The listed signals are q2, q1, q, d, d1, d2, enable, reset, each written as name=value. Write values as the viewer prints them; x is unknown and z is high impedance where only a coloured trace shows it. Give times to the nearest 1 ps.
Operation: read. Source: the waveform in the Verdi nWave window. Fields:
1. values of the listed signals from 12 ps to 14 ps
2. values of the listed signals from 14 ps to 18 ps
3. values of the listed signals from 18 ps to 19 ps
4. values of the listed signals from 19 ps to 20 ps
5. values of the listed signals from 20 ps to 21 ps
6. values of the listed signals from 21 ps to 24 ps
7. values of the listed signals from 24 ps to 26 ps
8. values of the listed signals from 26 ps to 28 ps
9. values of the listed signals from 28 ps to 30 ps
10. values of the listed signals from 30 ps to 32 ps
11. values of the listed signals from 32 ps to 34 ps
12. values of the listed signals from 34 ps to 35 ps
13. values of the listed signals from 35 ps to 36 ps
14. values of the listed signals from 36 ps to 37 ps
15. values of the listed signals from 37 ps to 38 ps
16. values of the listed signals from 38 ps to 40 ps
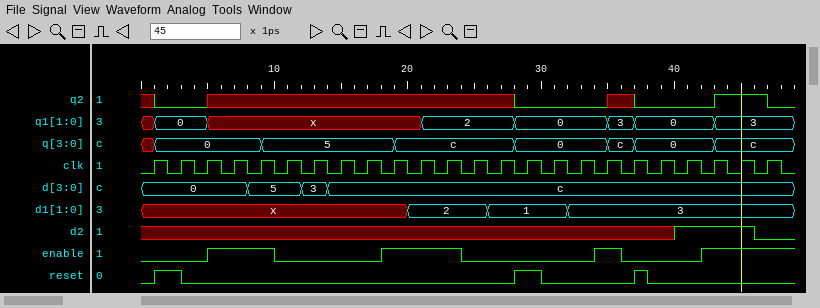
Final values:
q2=x, q1=x, q=5, d=3, d1=x, d2=x, enable=0, reset=0
q2=x, q1=x, q=5, d=c, d1=x, d2=x, enable=0, reset=0
q2=x, q1=x, q=5, d=c, d1=x, d2=x, enable=1, reset=0
q2=x, q1=x, q=c, d=c, d1=x, d2=x, enable=1, reset=0
q2=x, q1=x, q=c, d=c, d1=2, d2=x, enable=1, reset=0
q2=x, q1=2, q=c, d=c, d1=2, d2=x, enable=1, reset=0
q2=x, q1=2, q=c, d=c, d1=2, d2=x, enable=0, reset=0
q2=x, q1=2, q=c, d=c, d1=1, d2=x, enable=0, reset=0
q2=0, q1=0, q=0, d=c, d1=1, d2=x, enable=0, reset=1
q2=0, q1=0, q=0, d=c, d1=1, d2=x, enable=0, reset=0
q2=0, q1=0, q=0, d=c, d1=3, d2=x, enable=0, reset=0
q2=0, q1=0, q=0, d=c, d1=3, d2=x, enable=1, reset=0
q2=x, q1=3, q=c, d=c, d1=3, d2=x, enable=1, reset=0
q2=x, q1=3, q=c, d=c, d1=3, d2=x, enable=0, reset=0
q2=0, q1=0, q=0, d=c, d1=3, d2=x, enable=0, reset=1
q2=0, q1=0, q=0, d=c, d1=3, d2=x, enable=0, reset=0
